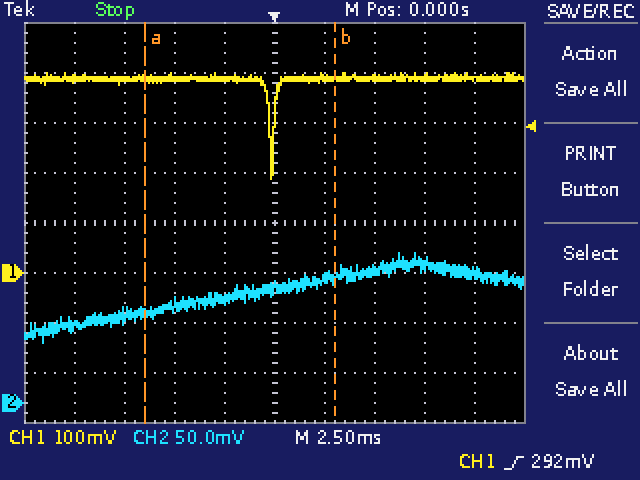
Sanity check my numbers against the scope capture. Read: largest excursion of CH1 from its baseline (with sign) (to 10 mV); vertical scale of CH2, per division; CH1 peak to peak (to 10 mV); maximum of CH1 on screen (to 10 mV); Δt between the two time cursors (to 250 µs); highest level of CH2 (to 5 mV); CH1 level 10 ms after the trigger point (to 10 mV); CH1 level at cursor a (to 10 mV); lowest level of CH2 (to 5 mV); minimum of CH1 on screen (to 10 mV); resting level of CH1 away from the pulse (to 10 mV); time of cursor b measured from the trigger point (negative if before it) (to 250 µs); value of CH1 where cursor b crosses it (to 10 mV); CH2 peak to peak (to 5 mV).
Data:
-200 mV
50 mV
210 mV
400 mV
9.50 ms
150 mV
390 mV
390 mV
60 mV
190 mV
390 mV
+3.00 ms
390 mV
90 mV
